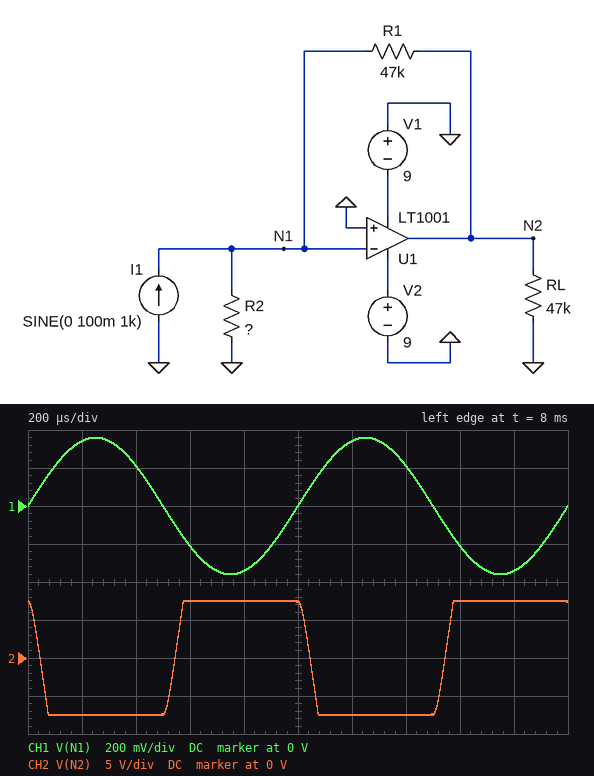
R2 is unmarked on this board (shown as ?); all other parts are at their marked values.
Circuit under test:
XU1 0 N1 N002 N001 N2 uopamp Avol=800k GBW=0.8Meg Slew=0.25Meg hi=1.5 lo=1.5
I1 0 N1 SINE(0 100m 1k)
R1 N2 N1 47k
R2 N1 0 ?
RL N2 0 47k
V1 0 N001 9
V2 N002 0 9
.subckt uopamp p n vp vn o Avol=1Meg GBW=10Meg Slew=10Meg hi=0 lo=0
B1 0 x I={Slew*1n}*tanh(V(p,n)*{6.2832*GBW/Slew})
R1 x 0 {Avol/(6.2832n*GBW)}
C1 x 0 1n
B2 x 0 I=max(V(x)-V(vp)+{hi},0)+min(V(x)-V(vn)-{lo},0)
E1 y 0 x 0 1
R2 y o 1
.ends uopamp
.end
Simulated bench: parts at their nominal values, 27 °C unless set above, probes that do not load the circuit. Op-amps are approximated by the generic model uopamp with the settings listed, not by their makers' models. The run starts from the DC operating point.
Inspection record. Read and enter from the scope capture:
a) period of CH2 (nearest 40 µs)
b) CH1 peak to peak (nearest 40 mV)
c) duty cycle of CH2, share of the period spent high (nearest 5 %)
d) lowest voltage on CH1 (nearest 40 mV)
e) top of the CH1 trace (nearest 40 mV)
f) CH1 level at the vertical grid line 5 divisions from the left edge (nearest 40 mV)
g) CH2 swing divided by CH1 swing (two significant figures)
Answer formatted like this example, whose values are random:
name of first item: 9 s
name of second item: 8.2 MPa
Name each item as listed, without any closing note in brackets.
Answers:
period of CH2: 1.00 ms
CH1 peak to peak: 720 mV
duty cycle of CH2, share of the period spent high: 50 %
lowest voltage on CH1: -360 mV
top of the CH1 trace: 360 mV
CH1 level at the vertical grid line 5 divisions from the left edge: 0 V
CH2 swing divided by CH1 swing: 21
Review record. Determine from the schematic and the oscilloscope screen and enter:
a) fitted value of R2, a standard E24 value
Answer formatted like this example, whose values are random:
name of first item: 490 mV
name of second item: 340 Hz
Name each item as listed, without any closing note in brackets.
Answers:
fitted value of R2, a standard E24 value: 3.6 Ω
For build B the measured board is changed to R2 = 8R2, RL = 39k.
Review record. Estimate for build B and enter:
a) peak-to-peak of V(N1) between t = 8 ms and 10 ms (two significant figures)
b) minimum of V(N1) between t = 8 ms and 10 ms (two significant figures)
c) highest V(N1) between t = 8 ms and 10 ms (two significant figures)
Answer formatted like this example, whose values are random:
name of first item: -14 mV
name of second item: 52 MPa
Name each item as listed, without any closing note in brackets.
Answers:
peak-to-peak of V(N1) between t = 8 ms and 10 ms: 1.6 V
minimum of V(N1) between t = 8 ms and 10 ms: -820 mV
highest V(N1) between t = 8 ms and 10 ms: 820 mV
